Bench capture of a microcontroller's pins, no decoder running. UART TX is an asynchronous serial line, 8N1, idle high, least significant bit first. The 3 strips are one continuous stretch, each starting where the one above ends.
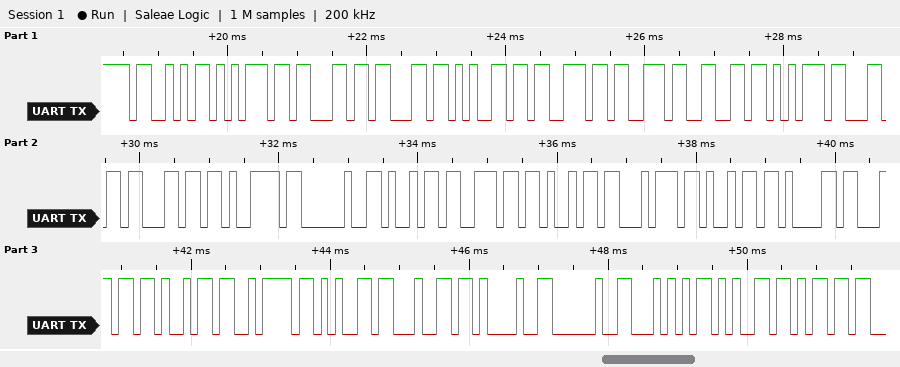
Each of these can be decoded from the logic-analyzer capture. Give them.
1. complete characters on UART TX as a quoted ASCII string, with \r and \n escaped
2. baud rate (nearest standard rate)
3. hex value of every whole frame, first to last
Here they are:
"Successfully initialized! Tem"
9600 baud
53 75 63 63 65 73 73 66 75 6C 6C 79 20 69 6E 69 74 69 61 6C 69 7A 65 64 21 20 54 65 6D
